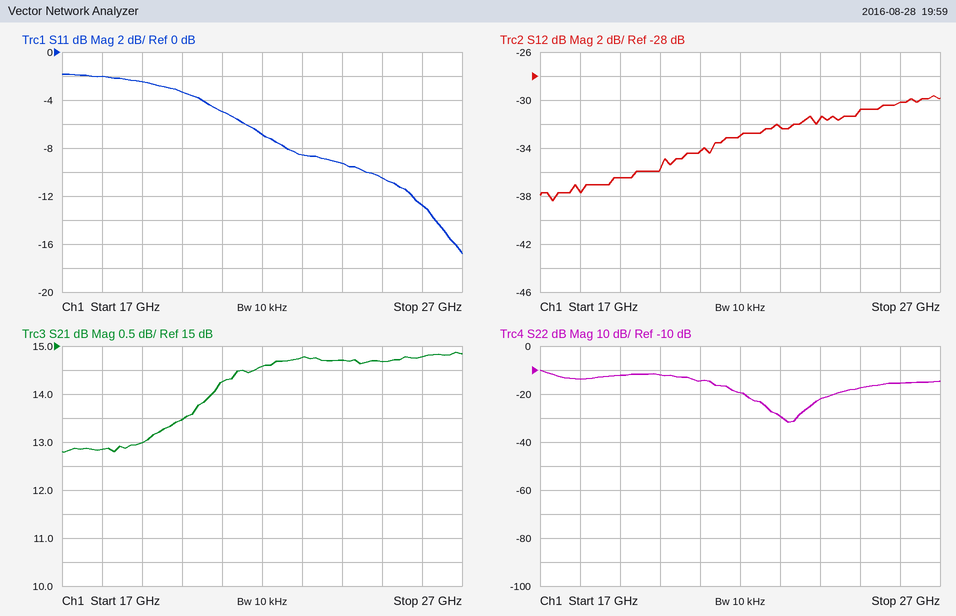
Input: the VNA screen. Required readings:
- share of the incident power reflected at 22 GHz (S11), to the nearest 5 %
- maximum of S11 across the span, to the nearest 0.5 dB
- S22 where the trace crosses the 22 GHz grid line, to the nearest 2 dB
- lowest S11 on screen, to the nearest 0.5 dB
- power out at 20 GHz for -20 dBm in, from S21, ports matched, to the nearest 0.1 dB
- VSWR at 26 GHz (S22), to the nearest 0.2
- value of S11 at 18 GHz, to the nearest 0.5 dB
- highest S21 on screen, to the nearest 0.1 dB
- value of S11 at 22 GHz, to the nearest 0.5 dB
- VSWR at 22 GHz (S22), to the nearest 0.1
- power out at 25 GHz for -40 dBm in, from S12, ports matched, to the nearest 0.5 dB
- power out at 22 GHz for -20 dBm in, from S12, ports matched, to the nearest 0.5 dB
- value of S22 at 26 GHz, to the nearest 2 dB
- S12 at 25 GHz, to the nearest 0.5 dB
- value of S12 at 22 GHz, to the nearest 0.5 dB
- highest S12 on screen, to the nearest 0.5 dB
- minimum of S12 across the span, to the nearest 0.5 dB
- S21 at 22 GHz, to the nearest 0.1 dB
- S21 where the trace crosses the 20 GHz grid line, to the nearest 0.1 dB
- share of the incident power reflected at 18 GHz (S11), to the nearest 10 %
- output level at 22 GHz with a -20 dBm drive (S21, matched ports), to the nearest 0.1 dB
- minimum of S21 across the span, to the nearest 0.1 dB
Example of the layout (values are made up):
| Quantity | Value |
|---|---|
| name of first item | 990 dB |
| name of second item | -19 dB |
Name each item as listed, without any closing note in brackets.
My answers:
| Quantity | Value |
|---|---|
| share of the incident power reflected at 22 GHz (S11), to the nearest 5 % | 20 % |
| maximum of S11 across the span, to the nearest 0.5 dB | -2.0 dB |
| S22 where the trace crosses the 22 GHz grid line, to the nearest 2 dB | -20 dB |
| lowest S11 on screen, to the nearest 0.5 dB | -17.0 dB |
| power out at 20 GHz for -20 dBm in, from S21, ports matched, to the nearest 0.1 dB | -6.5 dBm |
| VSWR at 26 GHz (S22), to the nearest 0.2 | 1.4 |
| value of S11 at 18 GHz, to the nearest 0.5 dB | -2.0 dB |
| highest S21 on screen, to the nearest 0.1 dB | 14.9 dB |
| value of S11 at 22 GHz, to the nearest 0.5 dB | -7.0 dB |
| VSWR at 22 GHz (S22), to the nearest 0.1 | 1.2 |
| power out at 25 GHz for -40 dBm in, from S12, ports matched, to the nearest 0.5 dB | -71.0 dBm |
| power out at 22 GHz for -20 dBm in, from S12, ports matched, to the nearest 0.5 dB | -53.0 dBm |
| value of S22 at 26 GHz, to the nearest 2 dB | -16 dB |
| S12 at 25 GHz, to the nearest 0.5 dB | -31.0 dB |
| value of S12 at 22 GHz, to the nearest 0.5 dB | -33.0 dB |
| highest S12 on screen, to the nearest 0.5 dB | -29.5 dB |
| minimum of S12 across the span, to the nearest 0.5 dB | -38.5 dB |
| S21 at 22 GHz, to the nearest 0.1 dB | 14.6 dB |
| S21 where the trace crosses the 20 GHz grid line, to the nearest 0.1 dB | 13.5 dB |
| share of the incident power reflected at 18 GHz (S11), to the nearest 10 % | 60 % |
| output level at 22 GHz with a -20 dBm drive (S21, matched ports), to the nearest 0.1 dB | -5.4 dBm |
| minimum of S21 across the span, to the nearest 0.1 dB | 12.8 dB |
